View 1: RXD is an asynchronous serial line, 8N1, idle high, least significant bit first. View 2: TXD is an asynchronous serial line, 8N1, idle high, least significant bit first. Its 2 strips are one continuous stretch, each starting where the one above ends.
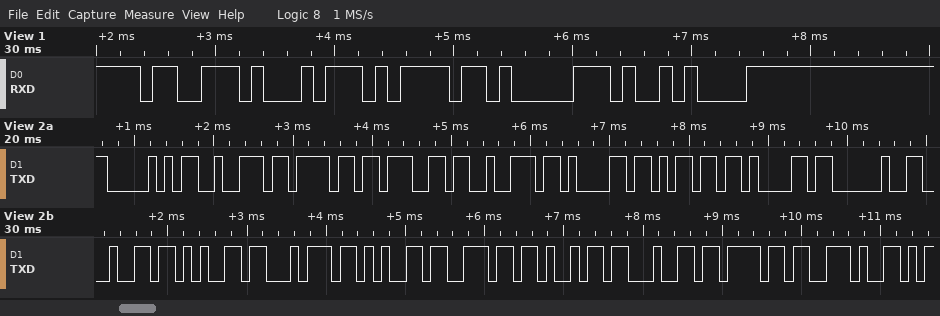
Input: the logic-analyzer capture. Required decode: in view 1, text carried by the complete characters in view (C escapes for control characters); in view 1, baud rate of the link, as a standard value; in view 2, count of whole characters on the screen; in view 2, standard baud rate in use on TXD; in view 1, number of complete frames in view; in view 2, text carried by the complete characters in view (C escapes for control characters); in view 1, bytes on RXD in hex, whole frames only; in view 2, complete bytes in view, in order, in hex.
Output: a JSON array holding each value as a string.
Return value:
["\"stop\\n\"", "9600 baud", "18", "9600 baud", "5", "\"Programa detenido.\"", "73 74 6F 70 0A", "50 72 6F 67 72 61 6D 61 20 64 65 74 65 6E 69 64 6F 2E"]
